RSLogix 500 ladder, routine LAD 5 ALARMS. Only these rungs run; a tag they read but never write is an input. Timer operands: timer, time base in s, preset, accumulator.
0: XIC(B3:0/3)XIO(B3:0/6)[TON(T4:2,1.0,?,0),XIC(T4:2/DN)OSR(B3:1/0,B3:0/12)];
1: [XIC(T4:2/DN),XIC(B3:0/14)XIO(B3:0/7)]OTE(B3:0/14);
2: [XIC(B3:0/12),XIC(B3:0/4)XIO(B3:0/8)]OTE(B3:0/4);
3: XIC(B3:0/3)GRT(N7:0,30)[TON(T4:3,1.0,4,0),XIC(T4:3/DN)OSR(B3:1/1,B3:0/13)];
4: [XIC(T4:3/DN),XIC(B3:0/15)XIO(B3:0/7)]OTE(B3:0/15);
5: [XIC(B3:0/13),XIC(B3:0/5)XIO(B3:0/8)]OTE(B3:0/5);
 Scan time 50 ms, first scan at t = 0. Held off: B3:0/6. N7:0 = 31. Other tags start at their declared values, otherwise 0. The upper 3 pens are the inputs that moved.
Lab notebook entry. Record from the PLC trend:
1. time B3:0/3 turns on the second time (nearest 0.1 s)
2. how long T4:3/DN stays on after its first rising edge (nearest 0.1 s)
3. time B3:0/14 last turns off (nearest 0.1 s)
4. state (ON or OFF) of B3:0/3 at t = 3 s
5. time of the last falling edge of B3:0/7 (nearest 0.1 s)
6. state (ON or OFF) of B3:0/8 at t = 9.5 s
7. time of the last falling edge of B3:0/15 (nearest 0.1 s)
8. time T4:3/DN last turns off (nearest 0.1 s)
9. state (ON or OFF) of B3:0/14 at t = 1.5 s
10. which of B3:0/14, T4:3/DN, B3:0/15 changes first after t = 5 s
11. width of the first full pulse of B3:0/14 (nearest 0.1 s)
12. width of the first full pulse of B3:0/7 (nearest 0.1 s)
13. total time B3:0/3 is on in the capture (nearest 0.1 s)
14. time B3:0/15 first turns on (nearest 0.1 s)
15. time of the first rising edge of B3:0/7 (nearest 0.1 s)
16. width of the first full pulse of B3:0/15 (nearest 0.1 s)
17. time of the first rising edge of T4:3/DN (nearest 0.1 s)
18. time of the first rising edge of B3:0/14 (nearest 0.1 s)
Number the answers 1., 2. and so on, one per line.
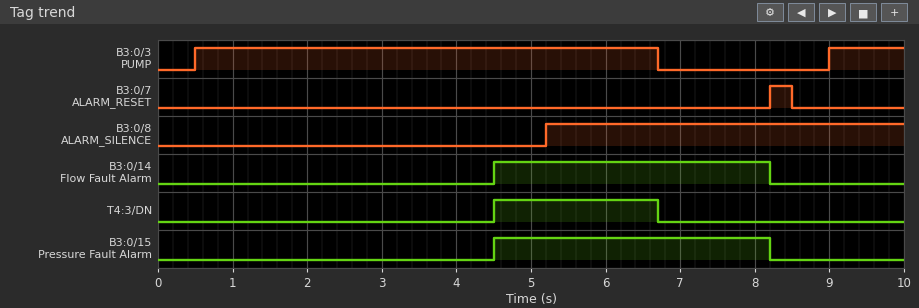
1. 9.0 s
2. 2.2 s
3. 8.2 s
4. ON
5. 8.5 s
6. ON
7. 8.2 s
8. 6.7 s
9. OFF
10. T4:3/DN
11. 3.7 s
12. 0.3 s
13. 7.2 s
14. 4.5 s
15. 8.2 s
16. 3.7 s
17. 4.5 s
18. 4.5 s
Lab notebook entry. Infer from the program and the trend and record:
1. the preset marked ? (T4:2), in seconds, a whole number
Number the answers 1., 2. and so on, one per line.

1. 4 s
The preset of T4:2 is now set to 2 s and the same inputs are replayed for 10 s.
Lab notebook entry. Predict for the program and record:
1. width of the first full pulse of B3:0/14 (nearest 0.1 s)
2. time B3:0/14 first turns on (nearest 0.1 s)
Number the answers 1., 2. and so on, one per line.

1. 5.7 s
2. 2.5 s
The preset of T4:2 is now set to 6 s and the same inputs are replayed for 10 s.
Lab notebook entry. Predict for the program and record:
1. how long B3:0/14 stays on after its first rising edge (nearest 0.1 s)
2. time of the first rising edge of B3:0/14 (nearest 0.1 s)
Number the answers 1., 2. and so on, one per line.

1. 1.7 s
2. 6.5 s
